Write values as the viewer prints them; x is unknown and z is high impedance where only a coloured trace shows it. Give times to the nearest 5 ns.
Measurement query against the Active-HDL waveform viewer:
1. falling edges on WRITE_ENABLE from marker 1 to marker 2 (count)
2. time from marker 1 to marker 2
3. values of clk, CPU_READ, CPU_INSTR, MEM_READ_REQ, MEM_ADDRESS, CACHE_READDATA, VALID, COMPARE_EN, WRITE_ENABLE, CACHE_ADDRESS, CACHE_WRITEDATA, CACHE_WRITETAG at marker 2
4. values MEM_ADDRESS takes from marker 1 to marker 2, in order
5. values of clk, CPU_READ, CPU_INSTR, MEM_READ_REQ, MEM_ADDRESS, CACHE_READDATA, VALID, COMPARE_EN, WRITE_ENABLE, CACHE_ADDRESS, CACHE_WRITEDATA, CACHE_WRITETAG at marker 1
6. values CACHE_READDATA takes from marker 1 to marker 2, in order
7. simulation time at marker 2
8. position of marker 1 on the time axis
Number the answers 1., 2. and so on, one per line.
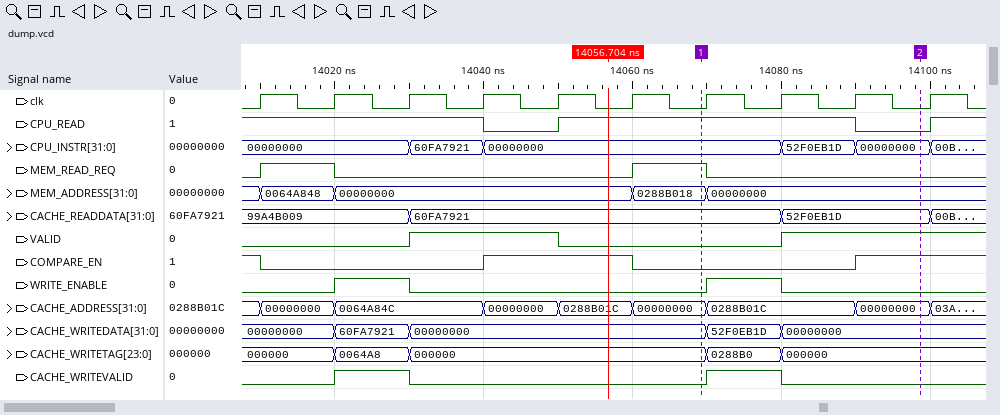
1. 1
2. 30 ns
3. clk=0, CPU_READ=0, CPU_INSTR=00000000, MEM_READ_REQ=0, MEM_ADDRESS=00000000, CACHE_READDATA=52F0EB1D, VALID=1, COMPARE_EN=1, WRITE_ENABLE=0, CACHE_ADDRESS=00000000, CACHE_WRITEDATA=00000000, CACHE_WRITETAG=000000
4. 0288B018, 00000000
5. clk=0, CPU_READ=1, CPU_INSTR=00000000, MEM_READ_REQ=1, MEM_ADDRESS=0288B018, CACHE_READDATA=60FA7921, VALID=0, COMPARE_EN=0, WRITE_ENABLE=0, CACHE_ADDRESS=00000000, CACHE_WRITEDATA=00000000, CACHE_WRITETAG=000000
6. 60FA7921, 52F0EB1D
7. 14100 ns
8. 14070 ns
